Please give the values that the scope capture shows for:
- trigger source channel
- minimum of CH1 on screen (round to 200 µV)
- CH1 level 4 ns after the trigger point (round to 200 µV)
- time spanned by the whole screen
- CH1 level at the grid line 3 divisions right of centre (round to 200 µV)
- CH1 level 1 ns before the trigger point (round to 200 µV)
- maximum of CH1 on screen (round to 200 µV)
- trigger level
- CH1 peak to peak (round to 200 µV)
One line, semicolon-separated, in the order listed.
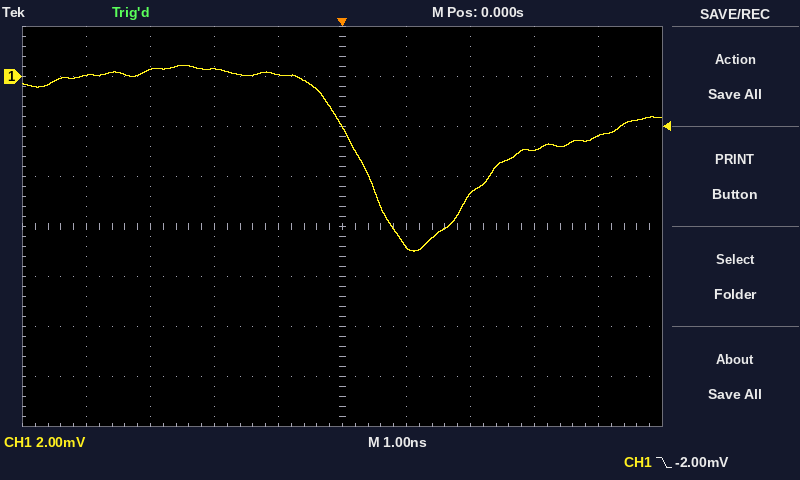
CH1; -7.0 mV; -2.4 mV; 10 ns; -3.0 mV; 0.0 mV; 400 µV; -2.00 mV; 7.4 mV
